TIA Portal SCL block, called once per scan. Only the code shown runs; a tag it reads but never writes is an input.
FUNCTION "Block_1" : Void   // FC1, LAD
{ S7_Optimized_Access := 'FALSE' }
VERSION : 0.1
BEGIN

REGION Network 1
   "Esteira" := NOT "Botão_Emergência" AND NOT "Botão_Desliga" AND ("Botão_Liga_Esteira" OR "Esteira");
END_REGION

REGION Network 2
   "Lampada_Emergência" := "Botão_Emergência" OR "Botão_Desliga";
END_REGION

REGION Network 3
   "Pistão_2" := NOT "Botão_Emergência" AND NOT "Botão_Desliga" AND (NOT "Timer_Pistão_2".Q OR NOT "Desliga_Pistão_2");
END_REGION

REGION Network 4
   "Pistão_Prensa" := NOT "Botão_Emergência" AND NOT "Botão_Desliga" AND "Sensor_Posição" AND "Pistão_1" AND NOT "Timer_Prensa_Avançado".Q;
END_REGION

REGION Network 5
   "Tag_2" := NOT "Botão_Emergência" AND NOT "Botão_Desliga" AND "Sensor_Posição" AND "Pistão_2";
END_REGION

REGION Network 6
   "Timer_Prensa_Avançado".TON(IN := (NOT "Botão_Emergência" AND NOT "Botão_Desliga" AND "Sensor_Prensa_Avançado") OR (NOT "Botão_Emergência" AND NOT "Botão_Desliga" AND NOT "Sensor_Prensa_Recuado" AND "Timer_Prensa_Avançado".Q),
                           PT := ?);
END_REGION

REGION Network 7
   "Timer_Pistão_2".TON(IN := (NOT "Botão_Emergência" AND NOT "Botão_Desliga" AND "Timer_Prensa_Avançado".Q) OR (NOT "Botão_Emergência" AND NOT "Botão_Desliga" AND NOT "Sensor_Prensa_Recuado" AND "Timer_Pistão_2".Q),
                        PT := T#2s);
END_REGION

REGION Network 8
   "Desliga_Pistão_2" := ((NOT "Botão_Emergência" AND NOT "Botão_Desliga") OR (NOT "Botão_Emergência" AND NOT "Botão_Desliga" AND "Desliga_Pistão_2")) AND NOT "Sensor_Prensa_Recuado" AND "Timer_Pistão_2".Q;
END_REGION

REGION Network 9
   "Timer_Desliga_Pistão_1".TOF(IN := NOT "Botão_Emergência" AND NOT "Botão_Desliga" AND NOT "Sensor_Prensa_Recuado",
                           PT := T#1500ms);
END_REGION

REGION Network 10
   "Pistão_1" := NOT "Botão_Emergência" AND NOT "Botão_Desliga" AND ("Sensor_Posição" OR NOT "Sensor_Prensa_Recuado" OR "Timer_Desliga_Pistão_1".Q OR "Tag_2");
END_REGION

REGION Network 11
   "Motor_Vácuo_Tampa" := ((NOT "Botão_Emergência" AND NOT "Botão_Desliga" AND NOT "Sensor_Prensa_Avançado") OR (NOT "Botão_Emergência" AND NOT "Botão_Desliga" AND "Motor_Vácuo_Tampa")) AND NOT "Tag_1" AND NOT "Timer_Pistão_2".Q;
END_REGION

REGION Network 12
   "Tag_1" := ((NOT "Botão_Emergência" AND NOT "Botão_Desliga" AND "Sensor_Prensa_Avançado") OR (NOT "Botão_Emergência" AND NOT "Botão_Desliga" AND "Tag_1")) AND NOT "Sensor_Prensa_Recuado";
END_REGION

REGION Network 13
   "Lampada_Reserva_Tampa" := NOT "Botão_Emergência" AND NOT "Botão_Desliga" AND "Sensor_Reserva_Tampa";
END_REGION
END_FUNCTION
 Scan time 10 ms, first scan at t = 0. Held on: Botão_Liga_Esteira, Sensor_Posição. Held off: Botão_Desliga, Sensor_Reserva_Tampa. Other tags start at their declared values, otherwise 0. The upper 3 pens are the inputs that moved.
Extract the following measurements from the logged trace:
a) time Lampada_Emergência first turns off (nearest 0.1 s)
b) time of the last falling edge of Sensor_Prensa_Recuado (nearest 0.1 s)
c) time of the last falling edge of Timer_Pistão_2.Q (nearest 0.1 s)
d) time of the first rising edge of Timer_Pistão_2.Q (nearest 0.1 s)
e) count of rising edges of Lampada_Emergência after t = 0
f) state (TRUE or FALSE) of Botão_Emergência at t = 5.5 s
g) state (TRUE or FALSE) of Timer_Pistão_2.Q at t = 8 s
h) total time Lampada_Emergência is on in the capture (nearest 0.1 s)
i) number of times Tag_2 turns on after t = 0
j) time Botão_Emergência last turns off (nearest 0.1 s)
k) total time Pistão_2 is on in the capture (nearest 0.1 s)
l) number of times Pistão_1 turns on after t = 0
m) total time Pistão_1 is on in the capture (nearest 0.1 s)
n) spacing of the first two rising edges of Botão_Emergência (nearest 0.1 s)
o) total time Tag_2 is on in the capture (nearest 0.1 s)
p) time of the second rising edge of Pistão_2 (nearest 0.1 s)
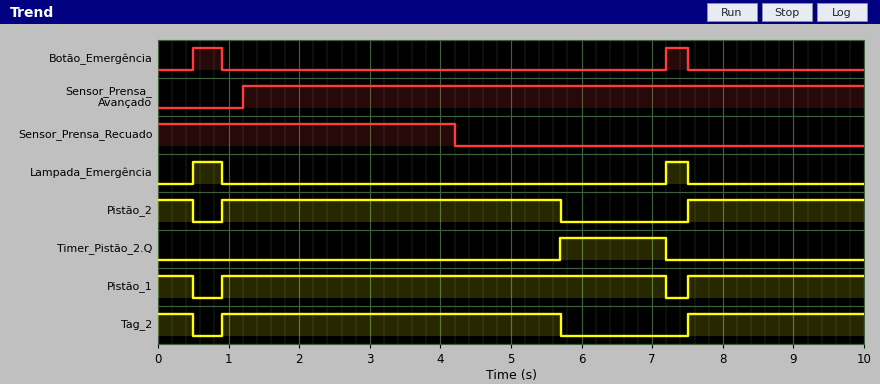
0.9 s
4.2 s
7.2 s
5.7 s
2
FALSE
FALSE
0.7 s
2
7.5 s
7.8 s
2
9.3 s
6.7 s
7.8 s
7.5 s
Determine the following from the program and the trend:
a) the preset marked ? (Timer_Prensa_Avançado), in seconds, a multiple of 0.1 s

2.5 s
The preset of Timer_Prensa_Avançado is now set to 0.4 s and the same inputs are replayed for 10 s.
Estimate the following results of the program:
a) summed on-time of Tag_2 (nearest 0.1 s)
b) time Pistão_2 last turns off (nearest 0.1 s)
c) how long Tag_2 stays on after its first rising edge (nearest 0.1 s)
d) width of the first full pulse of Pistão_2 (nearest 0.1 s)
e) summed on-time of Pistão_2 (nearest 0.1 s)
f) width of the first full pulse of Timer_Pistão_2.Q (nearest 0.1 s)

6.2 s
9.9 s
3.3 s
3.3 s
6.2 s
3.6 s
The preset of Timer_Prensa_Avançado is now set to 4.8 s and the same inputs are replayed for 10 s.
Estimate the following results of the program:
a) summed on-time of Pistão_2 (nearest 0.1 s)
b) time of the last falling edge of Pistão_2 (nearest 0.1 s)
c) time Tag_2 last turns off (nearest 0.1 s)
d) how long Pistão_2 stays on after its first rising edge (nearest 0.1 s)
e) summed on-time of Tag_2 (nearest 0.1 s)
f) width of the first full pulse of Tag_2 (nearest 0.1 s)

9.3 s
7.2 s
7.2 s
6.3 s
9.3 s
6.3 s
